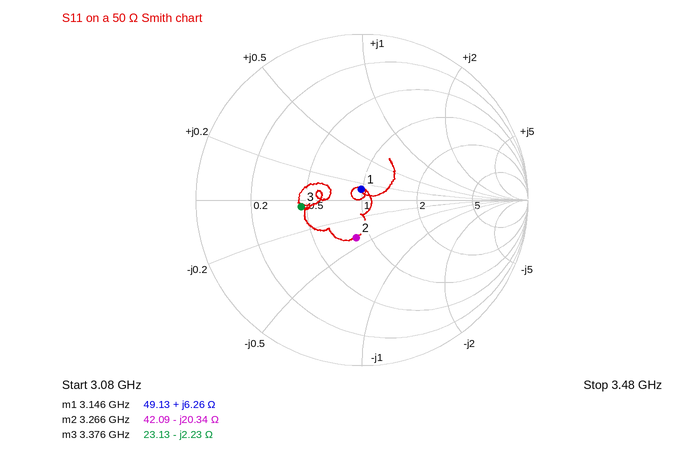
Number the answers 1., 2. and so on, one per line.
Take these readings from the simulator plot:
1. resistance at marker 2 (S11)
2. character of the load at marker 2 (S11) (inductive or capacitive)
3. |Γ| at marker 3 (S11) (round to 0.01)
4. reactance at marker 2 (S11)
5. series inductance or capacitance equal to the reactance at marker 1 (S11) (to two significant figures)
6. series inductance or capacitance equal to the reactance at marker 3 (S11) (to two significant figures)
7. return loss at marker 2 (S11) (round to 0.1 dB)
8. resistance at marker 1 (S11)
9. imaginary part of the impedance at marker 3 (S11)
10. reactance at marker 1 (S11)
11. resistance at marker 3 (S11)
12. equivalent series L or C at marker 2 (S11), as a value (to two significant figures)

1. 42.09 Ω
2. capacitive
3. 0.37
4. -20.34 Ω
5. 320 pH
6. 21 pF
7. 12.7 dB
8. 49.13 Ω
9. -2.23 Ω
10. +6.26 Ω
11. 23.13 Ω
12. 2.4 pF
